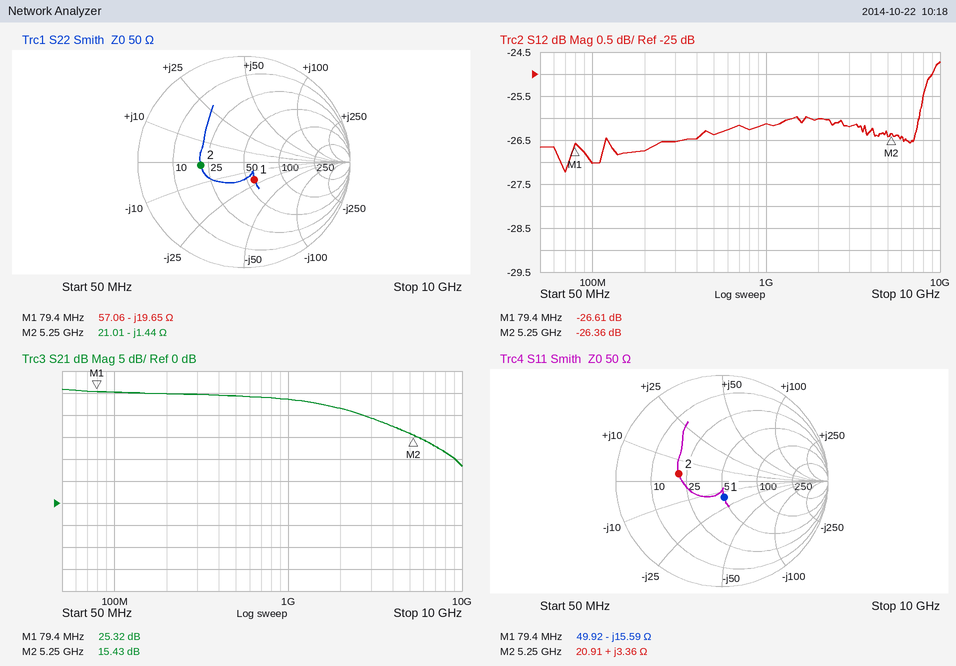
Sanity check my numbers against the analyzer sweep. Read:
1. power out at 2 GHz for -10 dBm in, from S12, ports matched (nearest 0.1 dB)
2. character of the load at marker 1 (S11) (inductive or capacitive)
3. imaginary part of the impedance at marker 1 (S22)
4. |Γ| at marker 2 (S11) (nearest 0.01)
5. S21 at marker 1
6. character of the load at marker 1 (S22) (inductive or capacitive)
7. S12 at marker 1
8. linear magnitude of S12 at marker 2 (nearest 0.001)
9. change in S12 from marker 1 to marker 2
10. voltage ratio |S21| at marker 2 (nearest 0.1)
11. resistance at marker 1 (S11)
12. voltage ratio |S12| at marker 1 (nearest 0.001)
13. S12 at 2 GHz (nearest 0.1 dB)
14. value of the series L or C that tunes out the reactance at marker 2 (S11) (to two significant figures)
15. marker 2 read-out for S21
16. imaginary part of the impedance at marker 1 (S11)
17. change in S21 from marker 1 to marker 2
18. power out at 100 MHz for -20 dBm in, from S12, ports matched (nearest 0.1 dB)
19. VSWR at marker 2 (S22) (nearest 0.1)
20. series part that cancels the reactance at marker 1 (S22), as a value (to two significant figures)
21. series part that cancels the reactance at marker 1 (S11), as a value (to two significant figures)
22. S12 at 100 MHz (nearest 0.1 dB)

-36.0 dBm
capacitive
-19.65 Ω
0.41
25.32 dB
capacitive
-26.61 dB
0.048
0.25 dB
5.9
49.92 Ω
0.047
-26.0 dB
9.0 pF
15.43 dB
-15.59 Ω
-9.89 dB
-47.0 dBm
2.4
39 nH
31 nH
-27.0 dB
